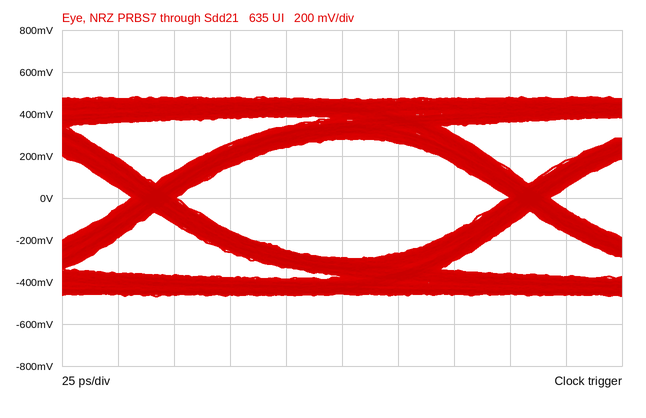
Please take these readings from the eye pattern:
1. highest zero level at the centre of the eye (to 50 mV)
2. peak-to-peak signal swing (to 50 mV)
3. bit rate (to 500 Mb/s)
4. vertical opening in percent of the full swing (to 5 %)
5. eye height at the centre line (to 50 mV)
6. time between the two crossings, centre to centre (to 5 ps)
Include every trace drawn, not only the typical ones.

-300 mV
950 mV
6.0 Gb/s
60 %
550 mV
165 ps
